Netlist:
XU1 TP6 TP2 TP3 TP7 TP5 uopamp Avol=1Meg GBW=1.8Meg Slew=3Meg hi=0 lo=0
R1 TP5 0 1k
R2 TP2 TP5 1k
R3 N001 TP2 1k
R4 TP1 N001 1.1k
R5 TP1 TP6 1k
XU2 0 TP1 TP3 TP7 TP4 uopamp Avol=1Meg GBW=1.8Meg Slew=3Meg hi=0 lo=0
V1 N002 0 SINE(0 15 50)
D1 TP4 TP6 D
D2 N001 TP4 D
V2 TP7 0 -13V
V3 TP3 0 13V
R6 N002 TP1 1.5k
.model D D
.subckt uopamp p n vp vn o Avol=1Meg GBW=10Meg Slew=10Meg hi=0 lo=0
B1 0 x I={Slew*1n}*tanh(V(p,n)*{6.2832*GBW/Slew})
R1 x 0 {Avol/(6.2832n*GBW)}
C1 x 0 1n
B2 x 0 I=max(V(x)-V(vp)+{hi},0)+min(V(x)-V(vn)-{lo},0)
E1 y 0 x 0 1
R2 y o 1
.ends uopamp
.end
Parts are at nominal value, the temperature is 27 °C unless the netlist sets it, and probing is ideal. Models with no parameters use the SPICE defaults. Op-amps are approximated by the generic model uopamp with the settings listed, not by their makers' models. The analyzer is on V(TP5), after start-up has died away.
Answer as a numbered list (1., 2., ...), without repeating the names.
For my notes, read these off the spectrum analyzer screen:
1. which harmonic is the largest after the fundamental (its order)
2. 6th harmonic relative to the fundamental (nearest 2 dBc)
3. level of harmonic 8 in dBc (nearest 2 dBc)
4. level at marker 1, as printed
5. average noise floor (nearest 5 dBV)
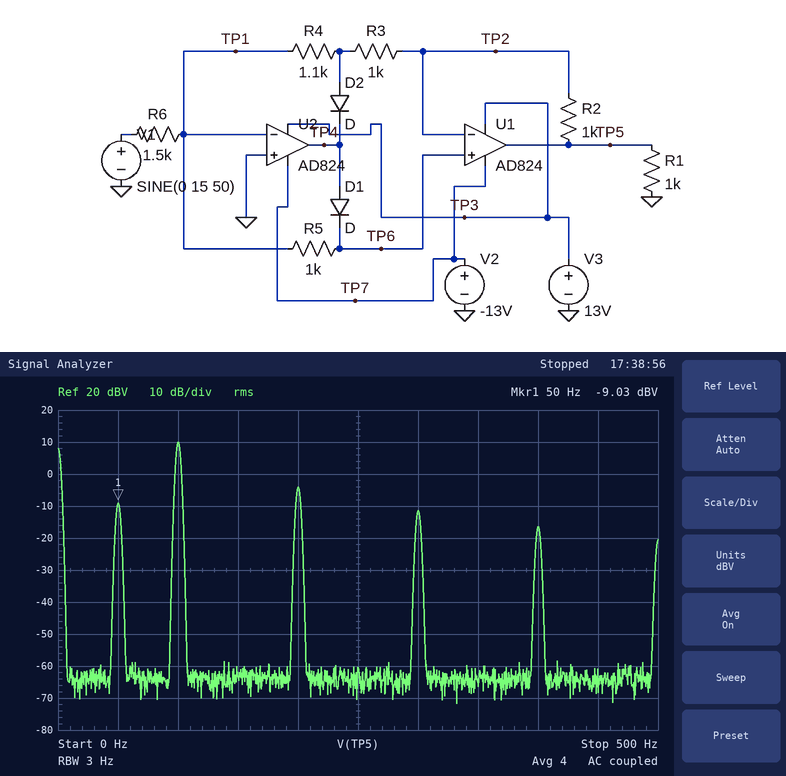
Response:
1. 2
2. -2 dBc
3. -8 dBc
4. -9.03 dBV
5. -65 dBV
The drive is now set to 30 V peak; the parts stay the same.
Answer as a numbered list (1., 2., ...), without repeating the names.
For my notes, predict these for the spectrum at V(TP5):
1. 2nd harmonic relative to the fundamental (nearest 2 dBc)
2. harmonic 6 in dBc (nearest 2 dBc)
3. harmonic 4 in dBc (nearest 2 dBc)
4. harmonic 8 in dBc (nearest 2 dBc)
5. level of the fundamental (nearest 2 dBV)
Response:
1. 32 dBc
2. 20 dBc
3. 28 dBc
4. 8 dBc
5. -22 dBV
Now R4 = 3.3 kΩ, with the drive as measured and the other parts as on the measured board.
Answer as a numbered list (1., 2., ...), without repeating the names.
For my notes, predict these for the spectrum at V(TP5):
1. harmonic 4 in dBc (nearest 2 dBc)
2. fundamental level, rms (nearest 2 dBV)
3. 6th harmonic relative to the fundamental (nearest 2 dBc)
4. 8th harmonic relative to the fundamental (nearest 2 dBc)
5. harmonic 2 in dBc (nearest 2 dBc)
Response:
1. -4 dBc
2. 6 dBV
3. -8 dBc
4. -12 dBc
5. 2 dBc
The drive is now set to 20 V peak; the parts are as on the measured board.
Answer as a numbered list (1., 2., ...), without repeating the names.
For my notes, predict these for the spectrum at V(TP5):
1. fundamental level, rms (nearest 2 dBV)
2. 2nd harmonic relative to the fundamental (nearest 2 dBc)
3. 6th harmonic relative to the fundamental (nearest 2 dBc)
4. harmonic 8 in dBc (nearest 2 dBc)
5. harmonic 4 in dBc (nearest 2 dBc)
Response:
1. -12 dBV
2. 24 dBc
3. 0 dBc
4. 0 dBc
5. 12 dBc
